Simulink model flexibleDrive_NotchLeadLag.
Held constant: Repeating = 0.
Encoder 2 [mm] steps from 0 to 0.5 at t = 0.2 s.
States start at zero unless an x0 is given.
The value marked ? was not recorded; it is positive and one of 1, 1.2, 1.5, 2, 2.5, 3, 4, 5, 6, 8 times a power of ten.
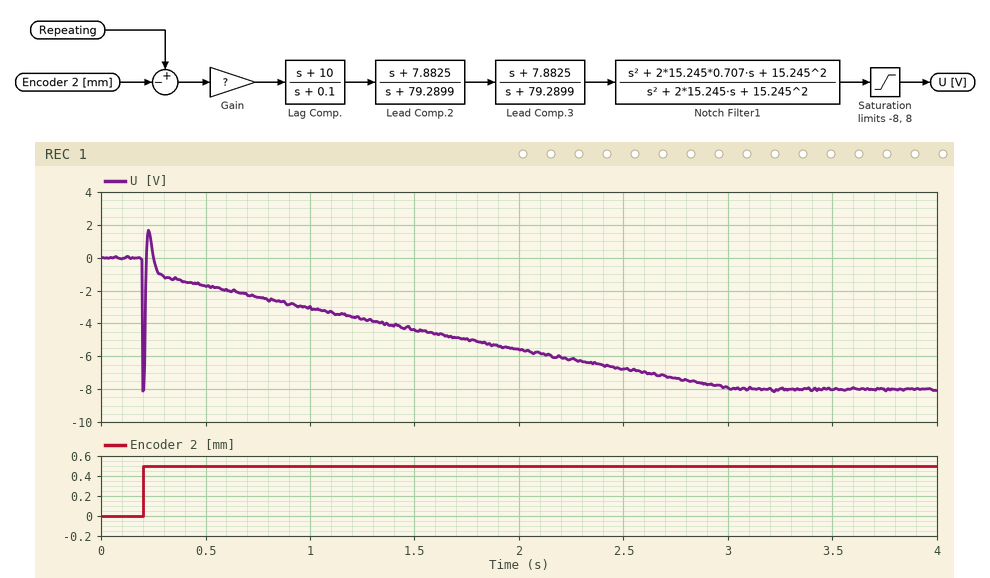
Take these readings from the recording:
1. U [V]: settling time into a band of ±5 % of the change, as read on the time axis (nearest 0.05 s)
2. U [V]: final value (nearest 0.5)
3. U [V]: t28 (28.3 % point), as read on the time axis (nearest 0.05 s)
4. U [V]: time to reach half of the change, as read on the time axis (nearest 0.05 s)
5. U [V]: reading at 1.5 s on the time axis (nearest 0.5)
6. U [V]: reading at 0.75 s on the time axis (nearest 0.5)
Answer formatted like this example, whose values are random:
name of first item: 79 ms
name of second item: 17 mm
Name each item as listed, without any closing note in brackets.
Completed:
U [V]: settling time into a band of ±5 % of the change, as read on the time axis: 2.85 s
U [V]: final value: -8.0
U [V]: t28 (28.3 % point), as read on the time axis: 0.20 s
U [V]: time to reach half of the change, as read on the time axis: 0.20 s
U [V]: reading at 1.5 s on the time axis: -4.5
U [V]: reading at 0.75 s on the time axis: -2.5
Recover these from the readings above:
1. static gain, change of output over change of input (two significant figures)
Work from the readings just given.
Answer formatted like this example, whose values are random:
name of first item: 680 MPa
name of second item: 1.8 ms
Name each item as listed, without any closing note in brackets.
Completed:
static gain, change of output over change of input: -16
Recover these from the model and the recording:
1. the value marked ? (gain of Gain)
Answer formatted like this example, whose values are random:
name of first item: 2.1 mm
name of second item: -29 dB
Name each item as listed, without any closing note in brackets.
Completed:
the value marked ?: 60
